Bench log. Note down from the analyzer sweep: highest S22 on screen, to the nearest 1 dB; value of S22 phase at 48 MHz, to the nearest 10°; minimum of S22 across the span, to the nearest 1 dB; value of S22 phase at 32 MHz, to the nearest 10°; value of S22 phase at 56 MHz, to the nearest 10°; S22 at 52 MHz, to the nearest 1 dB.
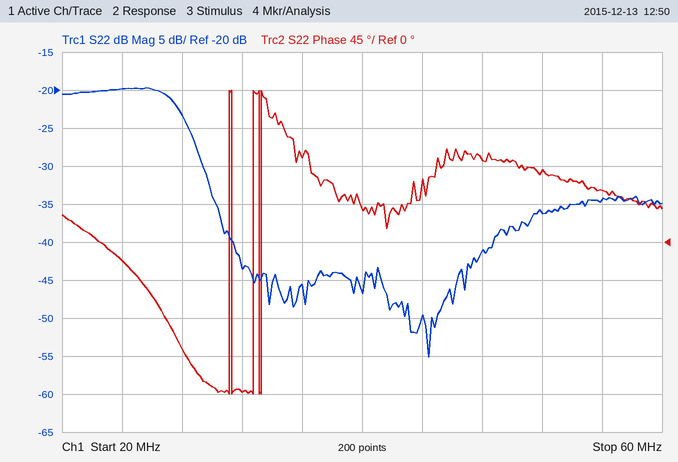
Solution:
-20 dB
100°
-55 dB
-180°
60°
-36 dB
